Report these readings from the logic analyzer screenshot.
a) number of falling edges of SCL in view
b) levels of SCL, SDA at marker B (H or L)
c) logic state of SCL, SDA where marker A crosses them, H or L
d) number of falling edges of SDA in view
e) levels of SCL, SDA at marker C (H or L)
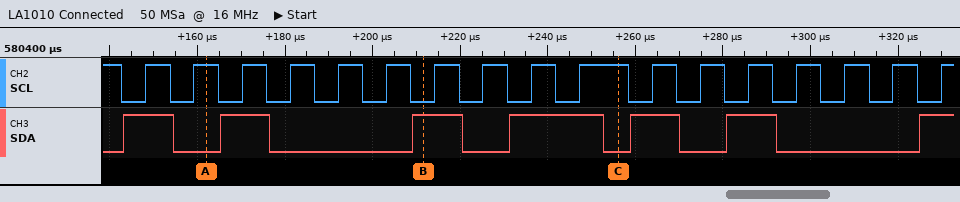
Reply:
17
SCL=L, SDA=H
SCL=H, SDA=L
6
SCL=H, SDA=L
